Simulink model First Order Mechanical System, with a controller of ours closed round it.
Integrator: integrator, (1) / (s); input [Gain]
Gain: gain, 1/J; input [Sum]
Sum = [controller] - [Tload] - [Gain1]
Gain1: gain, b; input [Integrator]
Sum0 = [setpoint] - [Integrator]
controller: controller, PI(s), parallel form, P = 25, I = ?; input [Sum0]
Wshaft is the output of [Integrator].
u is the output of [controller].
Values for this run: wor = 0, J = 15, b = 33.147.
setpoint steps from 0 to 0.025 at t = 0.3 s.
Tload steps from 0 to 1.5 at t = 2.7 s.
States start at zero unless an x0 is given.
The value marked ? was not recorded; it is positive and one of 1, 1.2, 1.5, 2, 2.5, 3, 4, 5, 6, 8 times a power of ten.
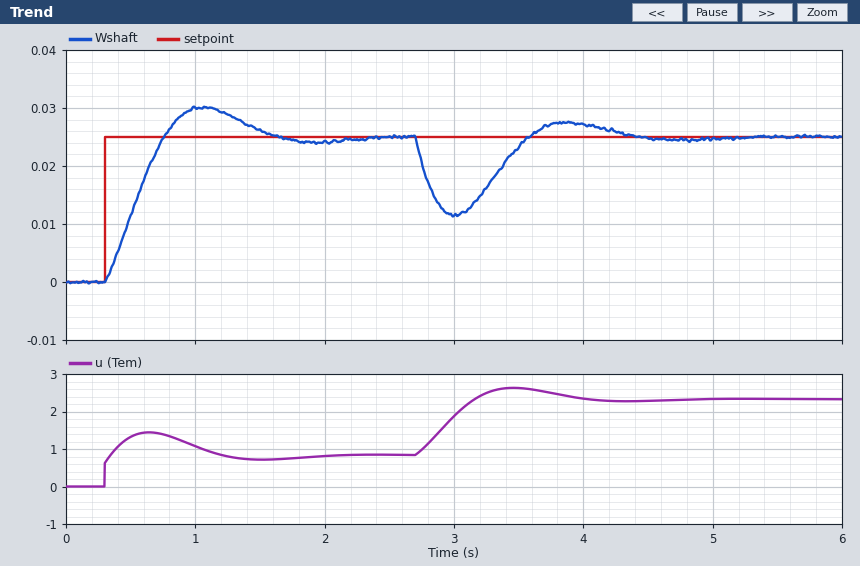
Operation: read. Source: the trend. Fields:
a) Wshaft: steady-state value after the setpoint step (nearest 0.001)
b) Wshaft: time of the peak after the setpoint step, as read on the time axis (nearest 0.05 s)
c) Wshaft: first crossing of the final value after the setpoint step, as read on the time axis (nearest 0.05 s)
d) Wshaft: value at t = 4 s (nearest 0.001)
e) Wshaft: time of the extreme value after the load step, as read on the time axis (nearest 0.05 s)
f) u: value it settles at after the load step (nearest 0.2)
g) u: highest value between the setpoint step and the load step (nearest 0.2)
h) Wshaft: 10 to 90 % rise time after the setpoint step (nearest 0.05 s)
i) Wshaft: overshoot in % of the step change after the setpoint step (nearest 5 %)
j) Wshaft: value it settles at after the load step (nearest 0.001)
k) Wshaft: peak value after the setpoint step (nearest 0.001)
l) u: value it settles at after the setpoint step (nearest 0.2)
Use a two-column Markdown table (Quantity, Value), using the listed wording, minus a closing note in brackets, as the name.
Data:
| Quantity | Value |
|---|---|
| Wshaft: steady-state value after the setpoint step | 0.025 |
| Wshaft: time of the peak after the setpoint step, as read on the time axis | 1.05 s |
| Wshaft: first crossing of the final value after the setpoint step, as read on the time axis | 0.75 s |
| Wshaft: value at t = 4 s | 0.027 |
| Wshaft: time of the extreme value after the load step, as read on the time axis | 3.00 s |
| u: value it settles at after the load step | 2.4 |
| u: highest value between the setpoint step and the load step | 1.4 |
| Wshaft: 10 to 90 % rise time after the setpoint step | 0.35 s |
| Wshaft: overshoot in % of the step change after the setpoint step | 20 % |
| Wshaft: value it settles at after the load step | 0.025 |
| Wshaft: peak value after the setpoint step | 0.030 |
| u: value it settles at after the setpoint step | 0.8 |
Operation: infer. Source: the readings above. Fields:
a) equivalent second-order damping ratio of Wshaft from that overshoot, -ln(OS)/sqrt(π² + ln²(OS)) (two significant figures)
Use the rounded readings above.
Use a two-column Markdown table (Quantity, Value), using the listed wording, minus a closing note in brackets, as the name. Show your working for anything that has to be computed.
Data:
| Quantity | Value |
|---|---|
| equivalent second-order damping ratio of Wshaft from that overshoot, -ln(OS)/sqrt(π² + ln²(OS)) | ln(0.2) = -1.609; 1.609 / sqrt(9.870 + 2.590) = 0.46 |
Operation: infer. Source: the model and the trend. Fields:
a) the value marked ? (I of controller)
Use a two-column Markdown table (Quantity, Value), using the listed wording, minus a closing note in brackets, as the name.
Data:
| Quantity | Value |
|---|---|
| the value marked ? | 250 |
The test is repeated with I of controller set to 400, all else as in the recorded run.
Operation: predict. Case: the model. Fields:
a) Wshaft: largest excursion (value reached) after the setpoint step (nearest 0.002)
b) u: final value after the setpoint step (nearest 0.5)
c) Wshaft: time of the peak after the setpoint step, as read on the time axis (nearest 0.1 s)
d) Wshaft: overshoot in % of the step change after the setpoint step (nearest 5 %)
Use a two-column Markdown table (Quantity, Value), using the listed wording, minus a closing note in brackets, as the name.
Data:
| Quantity | Value |
|---|---|
| Wshaft: largest excursion (value reached) after the setpoint step | 0.032 |
| u: final value after the setpoint step | 1.0 |
| Wshaft: time of the peak after the setpoint step, as read on the time axis | 0.9 s |
| Wshaft: overshoot in % of the step change after the setpoint step | 30 % |
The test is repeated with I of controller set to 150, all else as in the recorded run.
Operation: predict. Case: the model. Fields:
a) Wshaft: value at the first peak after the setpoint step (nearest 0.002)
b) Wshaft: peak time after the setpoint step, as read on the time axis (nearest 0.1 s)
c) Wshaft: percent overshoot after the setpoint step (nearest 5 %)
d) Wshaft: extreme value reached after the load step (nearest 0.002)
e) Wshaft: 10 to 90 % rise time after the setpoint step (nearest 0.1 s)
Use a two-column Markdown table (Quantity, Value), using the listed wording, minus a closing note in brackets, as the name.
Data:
| Quantity | Value |
|---|---|
| Wshaft: value at the first peak after the setpoint step | 0.028 |
| Wshaft: peak time after the setpoint step, as read on the time axis | 1.3 s |
| Wshaft: percent overshoot after the setpoint step | 10 % |
| Wshaft: extreme value reached after the load step | 0.010 |
| Wshaft: 10 to 90 % rise time after the setpoint step | 0.5 s |
